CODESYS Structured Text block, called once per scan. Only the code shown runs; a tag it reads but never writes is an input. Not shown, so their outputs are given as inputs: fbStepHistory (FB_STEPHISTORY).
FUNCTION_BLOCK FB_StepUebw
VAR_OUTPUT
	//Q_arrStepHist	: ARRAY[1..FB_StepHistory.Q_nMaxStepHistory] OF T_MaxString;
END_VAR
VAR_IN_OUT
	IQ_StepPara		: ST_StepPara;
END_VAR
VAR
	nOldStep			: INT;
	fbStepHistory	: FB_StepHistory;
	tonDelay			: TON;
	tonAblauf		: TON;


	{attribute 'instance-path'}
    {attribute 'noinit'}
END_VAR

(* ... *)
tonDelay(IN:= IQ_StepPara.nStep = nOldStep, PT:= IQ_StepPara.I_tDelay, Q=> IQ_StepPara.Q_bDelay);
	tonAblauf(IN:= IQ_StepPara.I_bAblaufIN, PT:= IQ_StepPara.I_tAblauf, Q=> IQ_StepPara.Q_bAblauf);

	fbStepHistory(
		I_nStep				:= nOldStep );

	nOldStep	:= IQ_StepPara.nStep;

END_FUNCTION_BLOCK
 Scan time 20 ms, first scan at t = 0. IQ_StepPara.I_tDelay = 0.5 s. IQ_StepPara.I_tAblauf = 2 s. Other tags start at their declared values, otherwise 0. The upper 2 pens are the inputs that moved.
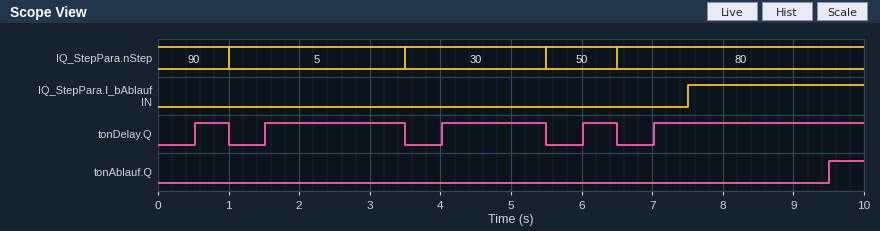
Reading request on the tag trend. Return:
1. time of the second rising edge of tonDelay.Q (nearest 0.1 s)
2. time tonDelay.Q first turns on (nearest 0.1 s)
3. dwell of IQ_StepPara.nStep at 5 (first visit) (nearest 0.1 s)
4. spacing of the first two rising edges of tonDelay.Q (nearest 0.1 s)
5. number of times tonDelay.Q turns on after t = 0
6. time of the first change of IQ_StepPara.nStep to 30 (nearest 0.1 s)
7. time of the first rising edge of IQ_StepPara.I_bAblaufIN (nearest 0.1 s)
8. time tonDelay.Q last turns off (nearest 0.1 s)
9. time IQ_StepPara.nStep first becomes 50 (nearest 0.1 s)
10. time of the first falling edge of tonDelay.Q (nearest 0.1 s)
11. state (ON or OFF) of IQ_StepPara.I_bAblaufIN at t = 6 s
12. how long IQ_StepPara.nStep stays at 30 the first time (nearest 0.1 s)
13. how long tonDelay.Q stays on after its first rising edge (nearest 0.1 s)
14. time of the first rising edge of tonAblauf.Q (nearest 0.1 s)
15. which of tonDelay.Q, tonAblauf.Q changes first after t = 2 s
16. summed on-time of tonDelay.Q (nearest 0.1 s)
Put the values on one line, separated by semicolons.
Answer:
1.5 s; 0.5 s; 2.5 s; 1.0 s; 5; 3.5 s; 7.5 s; 6.5 s; 5.5 s; 1.0 s; OFF; 2.0 s; 0.5 s; 9.5 s; tonDelay.Q; 7.4 s
